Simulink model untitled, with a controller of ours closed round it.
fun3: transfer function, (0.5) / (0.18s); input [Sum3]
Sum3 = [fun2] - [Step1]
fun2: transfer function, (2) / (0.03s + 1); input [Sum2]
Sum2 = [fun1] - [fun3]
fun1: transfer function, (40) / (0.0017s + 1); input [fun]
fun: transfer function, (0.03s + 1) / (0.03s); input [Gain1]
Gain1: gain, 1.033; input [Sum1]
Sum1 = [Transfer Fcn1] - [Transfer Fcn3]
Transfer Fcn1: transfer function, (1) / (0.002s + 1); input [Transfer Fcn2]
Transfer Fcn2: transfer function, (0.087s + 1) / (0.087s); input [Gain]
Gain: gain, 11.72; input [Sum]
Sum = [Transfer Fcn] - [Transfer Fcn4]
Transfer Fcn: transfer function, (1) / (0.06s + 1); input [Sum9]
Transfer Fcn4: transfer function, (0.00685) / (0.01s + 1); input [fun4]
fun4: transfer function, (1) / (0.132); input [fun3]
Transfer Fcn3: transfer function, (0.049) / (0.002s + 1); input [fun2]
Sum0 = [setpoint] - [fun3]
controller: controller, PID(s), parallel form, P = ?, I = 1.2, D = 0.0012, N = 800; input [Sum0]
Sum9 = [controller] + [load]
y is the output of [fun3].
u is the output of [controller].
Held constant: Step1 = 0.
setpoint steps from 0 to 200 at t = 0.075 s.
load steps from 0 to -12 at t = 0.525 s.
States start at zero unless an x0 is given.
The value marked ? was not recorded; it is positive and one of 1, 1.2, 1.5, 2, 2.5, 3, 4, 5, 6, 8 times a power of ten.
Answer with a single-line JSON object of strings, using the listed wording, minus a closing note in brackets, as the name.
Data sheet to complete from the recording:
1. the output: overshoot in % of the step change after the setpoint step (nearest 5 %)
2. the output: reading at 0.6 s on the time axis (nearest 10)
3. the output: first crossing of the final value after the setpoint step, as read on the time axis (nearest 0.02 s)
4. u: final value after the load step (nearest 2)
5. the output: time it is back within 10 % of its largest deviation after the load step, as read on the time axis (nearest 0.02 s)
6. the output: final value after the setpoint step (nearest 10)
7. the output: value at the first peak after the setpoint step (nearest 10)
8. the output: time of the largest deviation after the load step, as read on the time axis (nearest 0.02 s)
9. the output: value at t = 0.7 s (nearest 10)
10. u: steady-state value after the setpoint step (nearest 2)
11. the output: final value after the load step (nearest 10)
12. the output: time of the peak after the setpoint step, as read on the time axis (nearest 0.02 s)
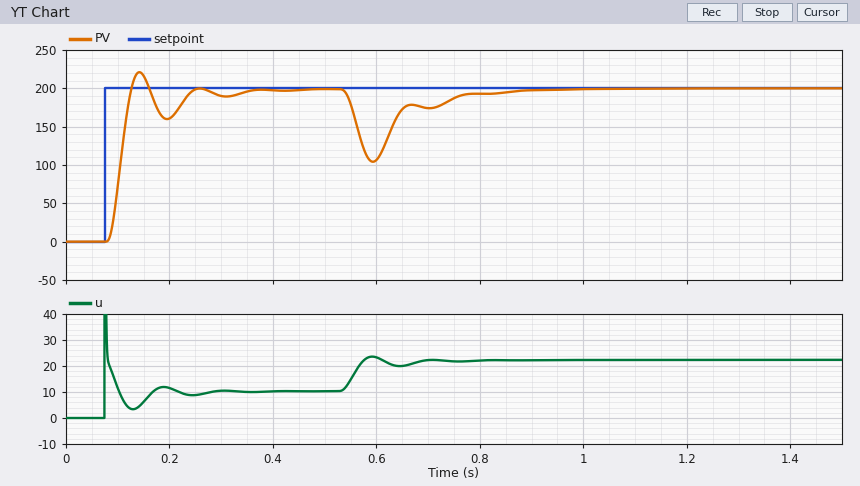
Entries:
{"the output: overshoot in % of the step change after the setpoint step": "10 %", "the output: reading at 0.6 s on the time axis": "110", "the output: first crossing of the final value after the setpoint step, as read on the time axis": "0.12 s", "u: final value after the load step": "22", "the output: time it is back within 10 % of its largest deviation after the load step, as read on the time axis": "0.76 s", "the output: final value after the setpoint step": "200", "the output: value at the first peak after the setpoint step": "220", "the output: time of the largest deviation after the load step, as read on the time axis": "0.60 s", "the output: value at t = 0.7 s": "170", "u: steady-state value after the setpoint step": "10", "the output: final value after the load step": "200", "the output: time of the peak after the setpoint step, as read on the time axis": "0.14 s"}
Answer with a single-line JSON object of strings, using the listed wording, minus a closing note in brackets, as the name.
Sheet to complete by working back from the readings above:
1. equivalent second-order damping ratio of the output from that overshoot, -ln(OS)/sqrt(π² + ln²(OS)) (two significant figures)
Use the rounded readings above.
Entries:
{"equivalent second-order damping ratio of the output from that overshoot, -ln(OS)/sqrt(π² + ln²(OS))": "0.59"}
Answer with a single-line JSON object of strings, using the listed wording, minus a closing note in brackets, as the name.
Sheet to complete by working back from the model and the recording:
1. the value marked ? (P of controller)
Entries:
{"the value marked ?": "0.1"}
